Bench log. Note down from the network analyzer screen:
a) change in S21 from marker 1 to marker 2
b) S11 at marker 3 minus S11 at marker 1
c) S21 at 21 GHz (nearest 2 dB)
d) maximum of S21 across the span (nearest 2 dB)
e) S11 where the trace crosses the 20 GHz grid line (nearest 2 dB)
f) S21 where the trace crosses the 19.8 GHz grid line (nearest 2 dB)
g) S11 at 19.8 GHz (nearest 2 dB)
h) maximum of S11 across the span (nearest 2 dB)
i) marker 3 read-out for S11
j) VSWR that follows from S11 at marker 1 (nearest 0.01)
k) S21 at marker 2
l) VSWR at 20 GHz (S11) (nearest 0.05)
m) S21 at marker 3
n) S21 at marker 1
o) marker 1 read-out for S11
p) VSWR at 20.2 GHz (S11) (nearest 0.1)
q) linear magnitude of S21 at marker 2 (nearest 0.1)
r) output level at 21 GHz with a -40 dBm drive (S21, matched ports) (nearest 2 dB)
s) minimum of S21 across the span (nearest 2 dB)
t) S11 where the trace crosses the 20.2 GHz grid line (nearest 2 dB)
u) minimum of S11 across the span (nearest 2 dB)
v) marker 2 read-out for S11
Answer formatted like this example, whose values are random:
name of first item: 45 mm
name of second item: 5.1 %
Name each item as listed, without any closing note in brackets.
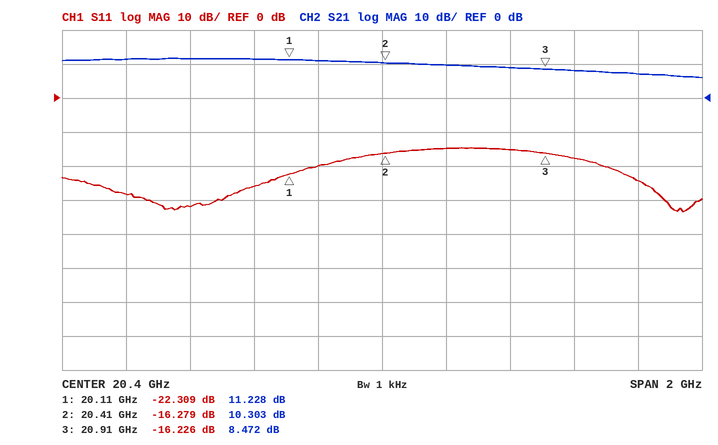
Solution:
change in S21 from marker 1 to marker 2: -0.925 dB
S11 at marker 3 minus S11 at marker 1: 6.083 dB
S21 at 21 GHz: 8 dB
maximum of S21 across the span: 12 dB
S11 where the trace crosses the 20 GHz grid line: -26 dB
S21 where the trace crosses the 19.8 GHz grid line: 12 dB
S11 at 19.8 GHz: -32 dB
maximum of S11 across the span: -14 dB
marker 3 read-out for S11: -16.226 dB
VSWR that follows from S11 at marker 1: 1.17
S21 at marker 2: 10.303 dB
VSWR at 20 GHz (S11): 1.10
S21 at marker 3: 8.472 dB
S21 at marker 1: 11.228 dB
marker 1 read-out for S11: -22.309 dB
VSWR at 20.2 GHz (S11): 1.2
linear magnitude of S21 at marker 2: 3.3
output level at 21 GHz with a -40 dBm drive (S21, matched ports): -32 dBm
minimum of S21 across the span: 6 dB
S11 where the trace crosses the 20.2 GHz grid line: -20 dB
minimum of S11 across the span: -34 dB
marker 2 read-out for S11: -16.279 dB
